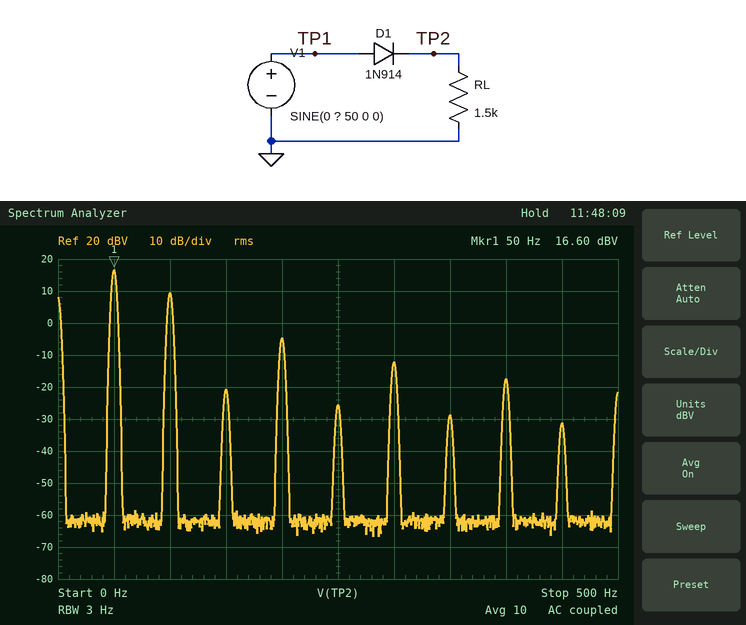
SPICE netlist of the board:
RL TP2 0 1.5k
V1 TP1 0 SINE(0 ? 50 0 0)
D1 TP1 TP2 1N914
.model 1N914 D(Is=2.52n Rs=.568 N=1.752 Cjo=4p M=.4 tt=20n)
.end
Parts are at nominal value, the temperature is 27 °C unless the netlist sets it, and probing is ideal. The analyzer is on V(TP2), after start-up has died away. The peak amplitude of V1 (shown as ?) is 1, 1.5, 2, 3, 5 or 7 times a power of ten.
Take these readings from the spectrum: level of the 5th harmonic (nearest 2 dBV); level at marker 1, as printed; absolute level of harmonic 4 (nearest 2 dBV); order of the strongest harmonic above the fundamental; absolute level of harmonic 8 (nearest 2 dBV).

-26 dBV
16.60 dBV
-4 dBV
2
-18 dBV
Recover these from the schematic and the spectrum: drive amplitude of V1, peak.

20 V
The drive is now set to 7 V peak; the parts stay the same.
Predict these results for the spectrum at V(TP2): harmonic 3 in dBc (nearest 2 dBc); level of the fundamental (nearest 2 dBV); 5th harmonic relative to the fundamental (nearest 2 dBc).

-28 dBc
6 dBV
-34 dBc
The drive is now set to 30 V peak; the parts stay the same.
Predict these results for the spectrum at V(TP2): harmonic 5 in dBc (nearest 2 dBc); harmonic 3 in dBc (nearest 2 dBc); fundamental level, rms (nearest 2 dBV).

-46 dBc
-40 dBc
20 dBV
